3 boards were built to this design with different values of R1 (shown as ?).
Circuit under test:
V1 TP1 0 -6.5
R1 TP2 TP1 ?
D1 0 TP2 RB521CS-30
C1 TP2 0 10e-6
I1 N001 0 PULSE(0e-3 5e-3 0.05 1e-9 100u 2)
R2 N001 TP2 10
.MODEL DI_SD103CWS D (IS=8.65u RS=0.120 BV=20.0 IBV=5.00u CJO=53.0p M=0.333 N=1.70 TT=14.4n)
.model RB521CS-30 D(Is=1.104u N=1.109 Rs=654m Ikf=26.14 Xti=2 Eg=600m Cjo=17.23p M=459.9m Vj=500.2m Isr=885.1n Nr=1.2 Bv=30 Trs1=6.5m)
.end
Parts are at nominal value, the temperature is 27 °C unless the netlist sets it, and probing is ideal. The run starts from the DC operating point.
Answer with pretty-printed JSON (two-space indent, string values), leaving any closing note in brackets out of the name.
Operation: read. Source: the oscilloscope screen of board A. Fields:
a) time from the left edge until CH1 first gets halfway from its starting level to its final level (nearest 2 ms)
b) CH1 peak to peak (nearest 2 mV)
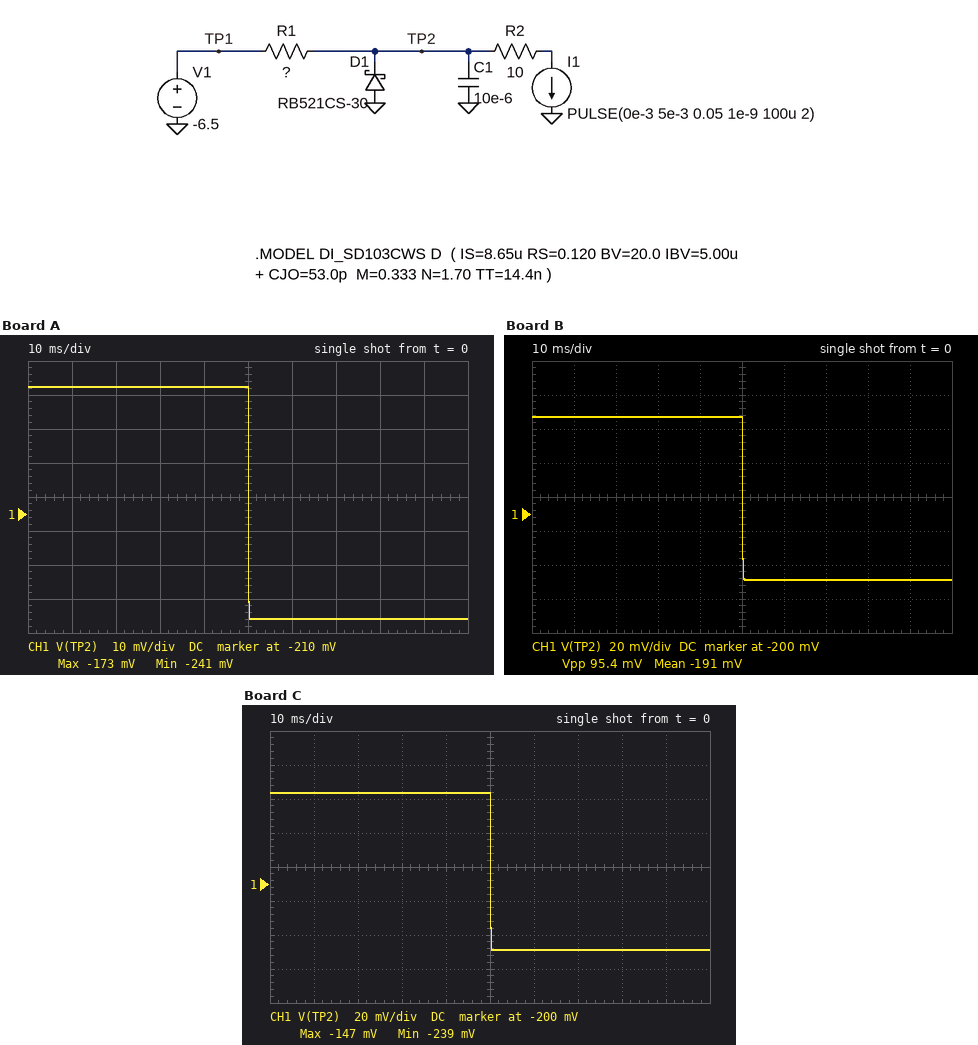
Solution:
{
  "time from the left edge until CH1 first gets halfway from its starting level to its final level": "50 ms",
  "CH1 peak to peak": "68 mV"
}
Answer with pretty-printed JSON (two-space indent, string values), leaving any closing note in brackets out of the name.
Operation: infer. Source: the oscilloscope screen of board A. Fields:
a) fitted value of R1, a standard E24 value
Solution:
{
  "fitted value of R1, a standard E24 value": "10 kΩ"
}
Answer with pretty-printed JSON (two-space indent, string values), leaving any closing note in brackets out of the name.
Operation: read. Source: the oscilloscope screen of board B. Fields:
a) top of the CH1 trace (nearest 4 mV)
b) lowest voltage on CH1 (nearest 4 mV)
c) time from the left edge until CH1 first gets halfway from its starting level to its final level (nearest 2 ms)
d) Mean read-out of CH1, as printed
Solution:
{
  "top of the CH1 trace": "-144 mV",
  "lowest voltage on CH1": "-240 mV",
  "time from the left edge until CH1 first gets halfway from its starting level to its final level": "50 ms",
  "Mean read-out of CH1, as printed": "-191 mV"
}
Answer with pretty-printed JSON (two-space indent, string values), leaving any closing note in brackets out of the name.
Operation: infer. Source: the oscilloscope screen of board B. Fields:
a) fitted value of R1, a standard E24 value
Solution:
{
  "fitted value of R1, a standard E24 value": "27 kΩ"
}
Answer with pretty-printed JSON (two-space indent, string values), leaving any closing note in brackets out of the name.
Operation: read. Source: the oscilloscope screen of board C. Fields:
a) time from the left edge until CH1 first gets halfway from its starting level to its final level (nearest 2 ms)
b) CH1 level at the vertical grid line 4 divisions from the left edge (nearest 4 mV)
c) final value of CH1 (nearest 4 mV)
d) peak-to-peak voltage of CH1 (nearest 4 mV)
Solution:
{
  "time from the left edge until CH1 first gets halfway from its starting level to its final level": "50 ms",
  "CH1 level at the vertical grid line 4 divisions from the left edge": "-148 mV",
  "final value of CH1": "-240 mV",
  "peak-to-peak voltage of CH1": "92 mV"
}
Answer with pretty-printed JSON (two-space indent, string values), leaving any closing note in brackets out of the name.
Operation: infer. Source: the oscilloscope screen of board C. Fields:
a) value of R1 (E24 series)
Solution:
{
  "value of R1": "24 kΩ"
}
